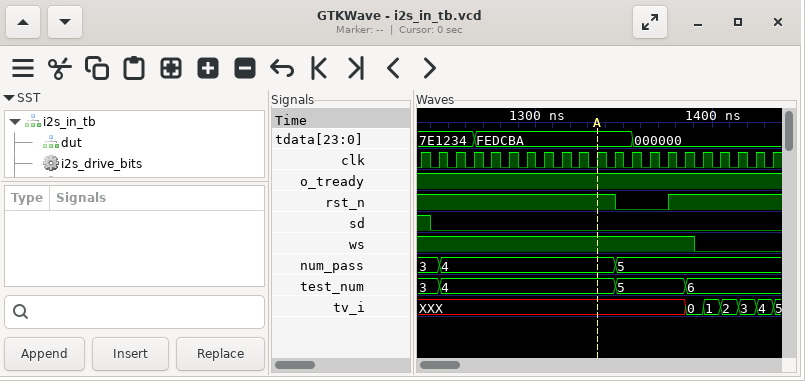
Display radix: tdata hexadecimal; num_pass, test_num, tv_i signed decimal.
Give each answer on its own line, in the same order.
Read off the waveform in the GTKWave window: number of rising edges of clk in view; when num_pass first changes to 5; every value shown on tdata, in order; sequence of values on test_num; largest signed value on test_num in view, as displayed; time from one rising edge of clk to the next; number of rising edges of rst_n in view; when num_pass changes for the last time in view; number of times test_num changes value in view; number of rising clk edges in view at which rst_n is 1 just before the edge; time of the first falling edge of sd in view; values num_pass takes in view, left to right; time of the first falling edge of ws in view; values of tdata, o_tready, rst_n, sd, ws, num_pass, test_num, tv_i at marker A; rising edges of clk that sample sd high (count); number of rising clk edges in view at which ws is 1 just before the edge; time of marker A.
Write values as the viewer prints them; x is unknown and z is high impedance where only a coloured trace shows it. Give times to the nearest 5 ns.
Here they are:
21
1345 ns
7E1234, FEDCBA, 000000
3, 4, 5, 6
6
10 ns
1
1345 ns
3
18
1240 ns
3, 4, 5
1390 ns
tdata=FEDCBA, o_tready=1, rst_n=1, sd=0, ws=1, num_pass=4, test_num=4, tv_i=XXX
1
16
1335 ns
